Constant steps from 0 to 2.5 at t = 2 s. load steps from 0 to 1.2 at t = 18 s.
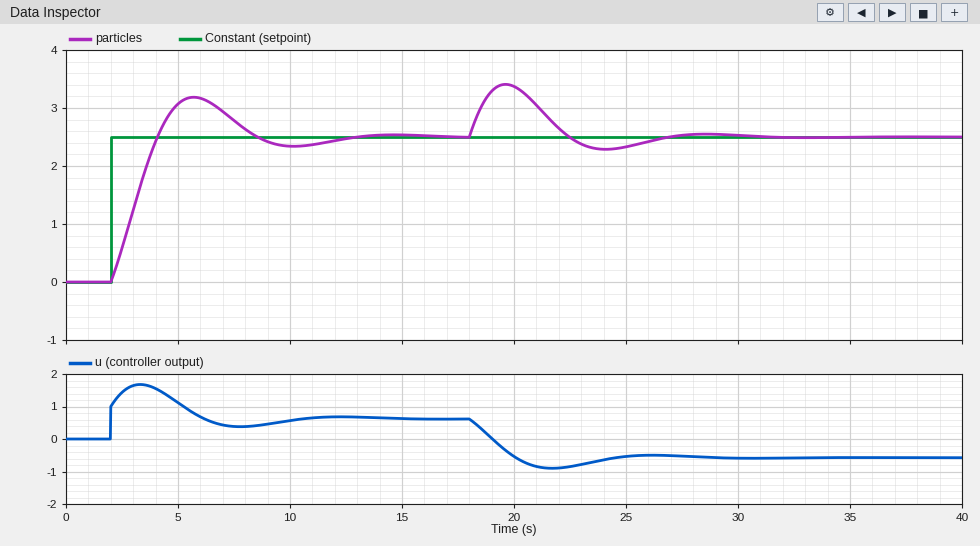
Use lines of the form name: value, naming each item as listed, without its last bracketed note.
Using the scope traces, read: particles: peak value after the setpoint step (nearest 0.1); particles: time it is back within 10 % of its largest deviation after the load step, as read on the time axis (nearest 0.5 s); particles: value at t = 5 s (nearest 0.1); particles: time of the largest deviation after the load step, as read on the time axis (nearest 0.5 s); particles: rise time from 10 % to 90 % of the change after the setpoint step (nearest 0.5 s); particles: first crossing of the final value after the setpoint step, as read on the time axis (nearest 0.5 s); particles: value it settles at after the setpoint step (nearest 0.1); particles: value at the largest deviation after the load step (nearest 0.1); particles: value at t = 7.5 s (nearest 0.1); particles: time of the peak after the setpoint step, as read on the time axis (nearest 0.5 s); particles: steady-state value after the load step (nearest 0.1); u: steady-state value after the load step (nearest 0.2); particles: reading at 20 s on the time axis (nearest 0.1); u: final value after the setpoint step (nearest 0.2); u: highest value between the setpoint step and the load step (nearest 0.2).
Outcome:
particles: peak value after the setpoint step: 3.2
particles: time it is back within 10 % of its largest deviation after the load step, as read on the time axis: 26.0 s
particles: value at t = 5 s: 3.1
particles: time of the largest deviation after the load step, as read on the time axis: 19.5 s
particles: rise time from 10 % to 90 % of the change after the setpoint step: 1.5 s
particles: first crossing of the final value after the setpoint step, as read on the time axis: 4.0 s
particles: value it settles at after the setpoint step: 2.5
particles: value at the largest deviation after the load step: 3.4
particles: value at t = 7.5 s: 2.8
particles: time of the peak after the setpoint step, as read on the time axis: 5.5 s
particles: steady-state value after the load step: 2.5
u: steady-state value after the load step: -0.6
particles: reading at 20 s on the time axis: 3.4
u: final value after the setpoint step: 0.6
u: highest value between the setpoint step and the load step: 1.6
